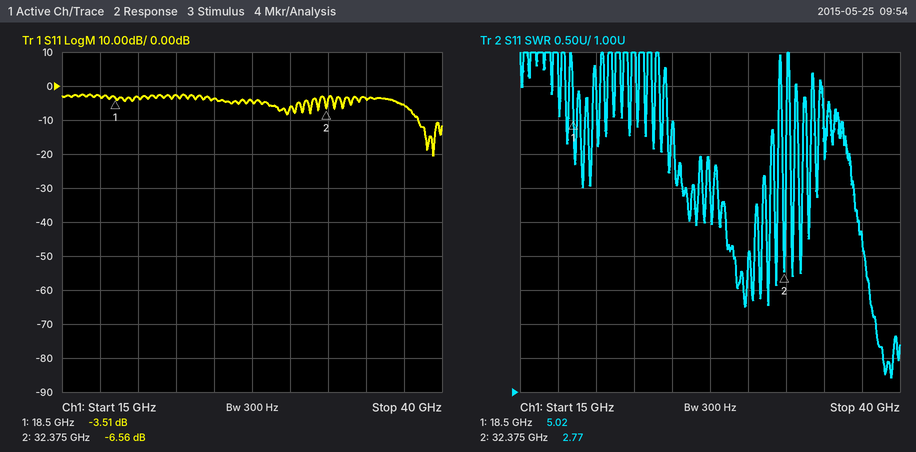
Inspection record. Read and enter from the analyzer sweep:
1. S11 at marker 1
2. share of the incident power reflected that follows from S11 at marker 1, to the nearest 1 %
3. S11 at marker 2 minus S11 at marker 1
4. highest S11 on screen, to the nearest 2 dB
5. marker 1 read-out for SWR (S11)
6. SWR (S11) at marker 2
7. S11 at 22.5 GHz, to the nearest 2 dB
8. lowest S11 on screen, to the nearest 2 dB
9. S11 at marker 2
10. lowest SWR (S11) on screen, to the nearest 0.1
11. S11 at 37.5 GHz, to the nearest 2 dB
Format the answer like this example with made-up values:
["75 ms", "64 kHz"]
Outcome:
["-3.51 dB", "45 %", "-3.05 dB", "-2 dB", "5.02", "2.77", "-2 dB", "-20 dB", "-6.56 dB", "1.2", "-6 dB"]
